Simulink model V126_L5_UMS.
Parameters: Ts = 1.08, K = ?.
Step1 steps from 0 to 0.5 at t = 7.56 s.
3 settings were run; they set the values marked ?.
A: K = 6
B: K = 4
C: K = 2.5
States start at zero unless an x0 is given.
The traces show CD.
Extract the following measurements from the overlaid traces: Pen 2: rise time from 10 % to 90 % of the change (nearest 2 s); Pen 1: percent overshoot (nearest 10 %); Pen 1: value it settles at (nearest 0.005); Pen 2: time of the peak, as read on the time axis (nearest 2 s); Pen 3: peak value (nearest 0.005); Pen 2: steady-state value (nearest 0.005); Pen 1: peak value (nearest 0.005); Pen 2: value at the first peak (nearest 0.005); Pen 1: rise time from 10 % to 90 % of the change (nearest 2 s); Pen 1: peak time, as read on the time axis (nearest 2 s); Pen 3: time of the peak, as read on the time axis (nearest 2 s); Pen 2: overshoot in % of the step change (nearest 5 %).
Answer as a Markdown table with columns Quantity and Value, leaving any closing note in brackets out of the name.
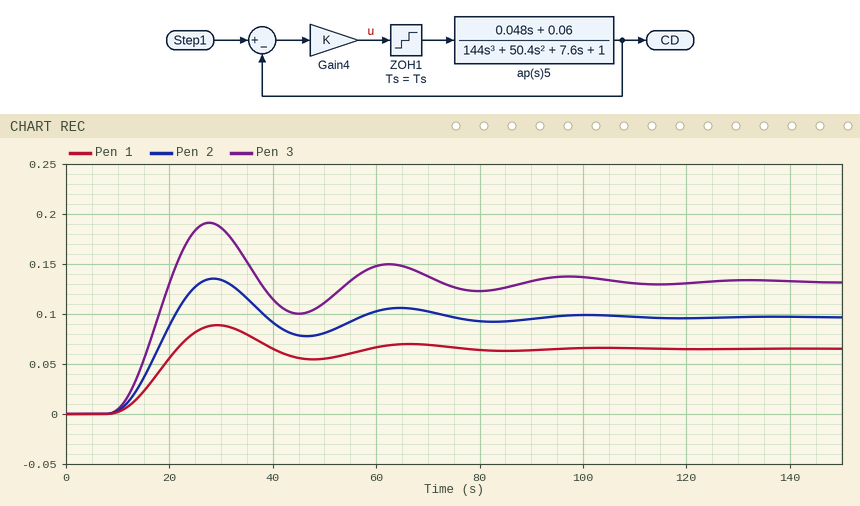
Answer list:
| Quantity | Value |
|---|---|
| Pen 2: rise time from 10 % to 90 % of the change | 8 s |
| Pen 1: percent overshoot | 40 % |
| Pen 1: value it settles at | 0.065 |
| Pen 2: time of the peak, as read on the time axis | 28 s |
| Pen 3: peak value | 0.190 |
| Pen 2: steady-state value | 0.095 |
| Pen 1: peak value | 0.090 |
| Pen 2: value at the first peak | 0.135 |
| Pen 1: rise time from 10 % to 90 % of the change | 8 s |
| Pen 1: peak time, as read on the time axis | 30 s |
| Pen 3: time of the peak, as read on the time axis | 28 s |
| Pen 2: overshoot in % of the step change | 40 % |
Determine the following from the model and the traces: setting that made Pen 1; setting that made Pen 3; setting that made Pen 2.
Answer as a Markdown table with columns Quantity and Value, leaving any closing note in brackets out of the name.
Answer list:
| Quantity | Value |
|---|---|
| setting that made Pen 1 | C |
| setting that made Pen 3 | A |
| setting that made Pen 2 | B |
